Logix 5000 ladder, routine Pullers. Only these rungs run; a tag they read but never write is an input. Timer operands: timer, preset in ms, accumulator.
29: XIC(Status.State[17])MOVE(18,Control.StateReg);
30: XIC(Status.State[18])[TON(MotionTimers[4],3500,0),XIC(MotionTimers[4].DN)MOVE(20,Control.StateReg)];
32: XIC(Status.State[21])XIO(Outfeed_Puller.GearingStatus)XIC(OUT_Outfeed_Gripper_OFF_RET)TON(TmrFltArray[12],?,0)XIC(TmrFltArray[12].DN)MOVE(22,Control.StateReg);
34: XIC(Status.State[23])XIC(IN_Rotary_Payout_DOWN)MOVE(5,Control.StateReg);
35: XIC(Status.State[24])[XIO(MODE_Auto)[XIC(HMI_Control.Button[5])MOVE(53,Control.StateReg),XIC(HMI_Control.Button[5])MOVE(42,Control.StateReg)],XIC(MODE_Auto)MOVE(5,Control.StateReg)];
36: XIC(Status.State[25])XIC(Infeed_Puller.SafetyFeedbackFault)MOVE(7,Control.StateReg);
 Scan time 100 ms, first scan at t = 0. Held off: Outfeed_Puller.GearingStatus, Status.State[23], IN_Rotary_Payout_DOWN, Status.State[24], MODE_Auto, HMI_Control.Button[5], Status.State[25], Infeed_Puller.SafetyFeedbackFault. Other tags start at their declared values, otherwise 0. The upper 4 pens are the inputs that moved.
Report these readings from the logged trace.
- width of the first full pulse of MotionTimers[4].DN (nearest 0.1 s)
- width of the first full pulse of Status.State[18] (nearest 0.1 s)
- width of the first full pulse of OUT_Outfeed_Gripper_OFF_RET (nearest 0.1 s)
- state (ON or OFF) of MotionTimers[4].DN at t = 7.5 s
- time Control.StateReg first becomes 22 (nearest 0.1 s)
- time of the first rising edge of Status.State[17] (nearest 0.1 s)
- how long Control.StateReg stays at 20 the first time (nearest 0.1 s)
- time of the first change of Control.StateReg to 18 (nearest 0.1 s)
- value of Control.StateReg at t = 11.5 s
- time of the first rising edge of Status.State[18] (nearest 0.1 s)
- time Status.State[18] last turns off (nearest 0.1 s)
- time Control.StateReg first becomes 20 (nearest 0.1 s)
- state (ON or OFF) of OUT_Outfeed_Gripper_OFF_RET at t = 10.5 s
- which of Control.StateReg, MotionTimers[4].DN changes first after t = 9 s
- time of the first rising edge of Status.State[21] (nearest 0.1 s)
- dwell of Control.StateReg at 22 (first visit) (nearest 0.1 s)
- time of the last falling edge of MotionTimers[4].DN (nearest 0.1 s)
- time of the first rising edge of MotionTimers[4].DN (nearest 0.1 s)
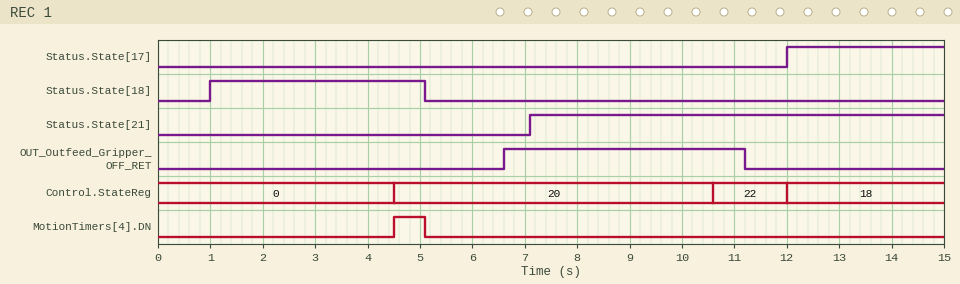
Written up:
0.6 s
4.1 s
4.6 s
OFF
10.6 s
12.0 s
6.1 s
12.0 s
22
1.0 s
5.1 s
4.5 s
ON
Control.StateReg
7.1 s
1.4 s
5.1 s
4.5 s
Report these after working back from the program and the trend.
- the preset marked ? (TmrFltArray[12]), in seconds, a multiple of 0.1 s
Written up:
3.5 s
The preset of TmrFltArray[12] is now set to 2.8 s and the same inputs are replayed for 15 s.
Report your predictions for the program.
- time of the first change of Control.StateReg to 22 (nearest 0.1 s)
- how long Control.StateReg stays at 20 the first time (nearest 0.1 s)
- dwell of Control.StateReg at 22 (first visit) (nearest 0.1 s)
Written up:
9.9 s
5.4 s
2.1 s
